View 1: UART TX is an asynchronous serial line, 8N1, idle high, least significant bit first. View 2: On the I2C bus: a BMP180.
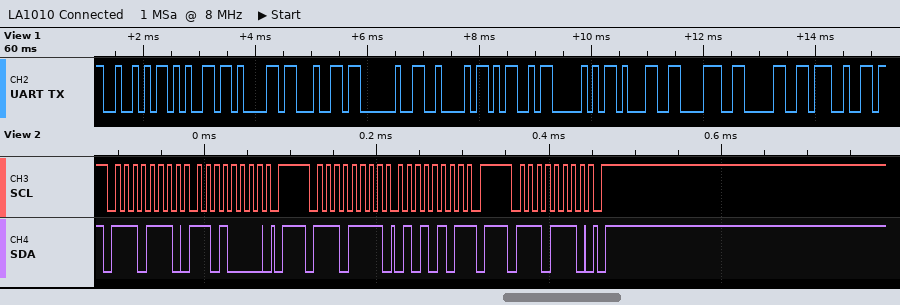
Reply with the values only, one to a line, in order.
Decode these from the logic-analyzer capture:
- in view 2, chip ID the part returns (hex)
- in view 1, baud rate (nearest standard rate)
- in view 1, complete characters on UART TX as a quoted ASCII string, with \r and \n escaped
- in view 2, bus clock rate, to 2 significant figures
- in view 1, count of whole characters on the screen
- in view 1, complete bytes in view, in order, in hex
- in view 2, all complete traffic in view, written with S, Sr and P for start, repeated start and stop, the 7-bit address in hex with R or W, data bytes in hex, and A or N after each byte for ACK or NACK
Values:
0x55
9600 baud
"Read BMP180'"
100 kHz
12
0x52 0x65 0x61 0x64 0x20 0x42 0x4D 0x50 0x31 0x38 0x30 0x27
S 77W A D0 A P S 77R A 55 N P S 77W A P
